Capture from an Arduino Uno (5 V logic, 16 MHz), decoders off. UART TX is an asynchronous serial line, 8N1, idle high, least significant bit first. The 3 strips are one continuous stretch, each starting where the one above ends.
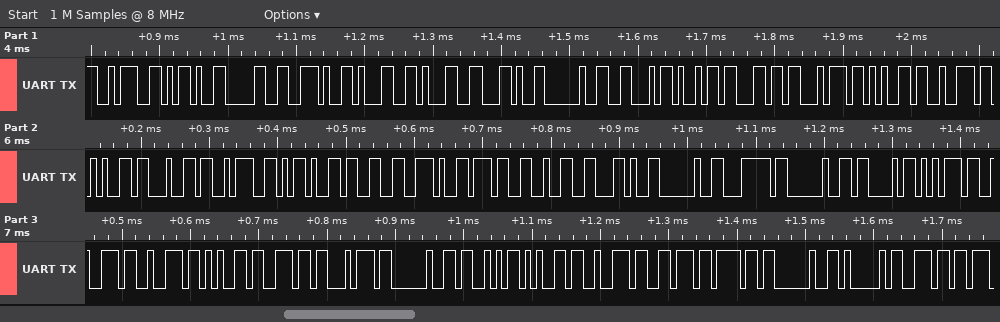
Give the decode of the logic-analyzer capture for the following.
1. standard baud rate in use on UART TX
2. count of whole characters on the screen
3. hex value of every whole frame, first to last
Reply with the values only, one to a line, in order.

115200 baud
42
3A 2D 30 2E 31 31 2C 20 46 69 6C 74 65 72 65 64 3A 2D 33 2E 37 32 2C 20 7C 20 43 75 72 72 65 6E 74 20 53 65 72 76 6F 20 41 6E
